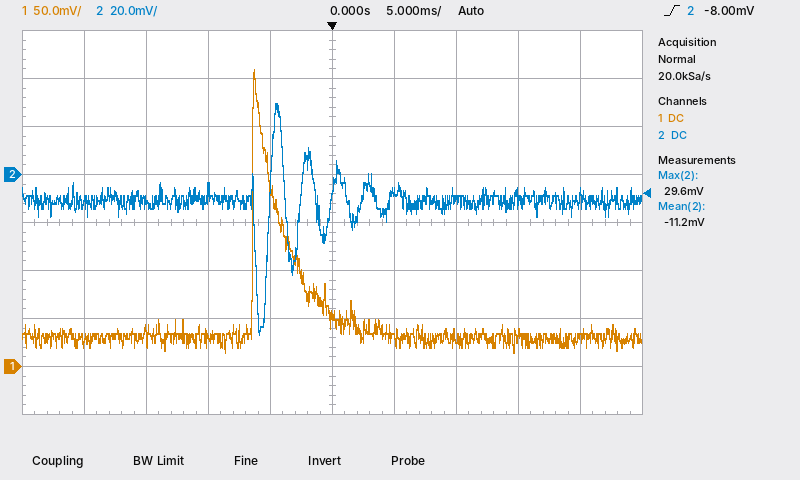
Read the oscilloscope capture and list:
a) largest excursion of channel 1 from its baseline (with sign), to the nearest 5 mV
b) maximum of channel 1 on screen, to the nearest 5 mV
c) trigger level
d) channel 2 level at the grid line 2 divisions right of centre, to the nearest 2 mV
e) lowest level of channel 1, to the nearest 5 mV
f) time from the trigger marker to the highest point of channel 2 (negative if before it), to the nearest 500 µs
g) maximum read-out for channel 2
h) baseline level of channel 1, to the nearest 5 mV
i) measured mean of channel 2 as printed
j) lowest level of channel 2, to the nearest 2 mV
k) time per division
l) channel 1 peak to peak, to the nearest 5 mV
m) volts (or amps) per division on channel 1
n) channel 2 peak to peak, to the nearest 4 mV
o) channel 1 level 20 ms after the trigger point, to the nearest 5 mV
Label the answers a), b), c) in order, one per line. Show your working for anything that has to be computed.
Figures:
a) 310 mV − (30 mV) = +280 mV
b) 310 mV
c) -8.00 mV
d) -10 mV
e) 15 mV
f) -4.5 ms
g) 29.6 mV
h) 30 mV
i) -11.2 mV
j) -66 mV
k) 5 ms
l) 310 mV − (15 mV) = 295 mV
m) 50 mV
n) 96 mV
o) 30 mV
